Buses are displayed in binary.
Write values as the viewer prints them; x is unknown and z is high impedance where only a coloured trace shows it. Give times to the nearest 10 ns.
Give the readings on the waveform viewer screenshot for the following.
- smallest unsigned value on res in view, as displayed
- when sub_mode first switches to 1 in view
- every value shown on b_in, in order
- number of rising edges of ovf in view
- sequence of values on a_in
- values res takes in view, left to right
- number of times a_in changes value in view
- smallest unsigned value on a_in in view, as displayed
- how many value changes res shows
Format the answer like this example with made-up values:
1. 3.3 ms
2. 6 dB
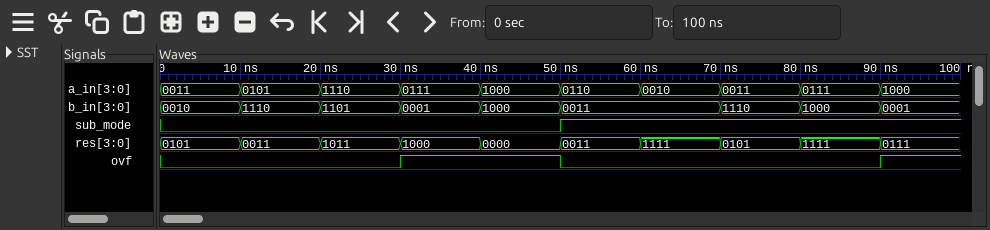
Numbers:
1. 0000
2. 50 ns
3. 0010, 1110, 1101, 0001, 1000, 0011, 1110, 1000, 0001
4. 2
5. 0011, 0101, 1110, 0111, 1000, 0110, 0010, 0011, 0111, 1000
6. 0101, 0011, 1011, 1000, 0000, 0011, 1111, 0101, 1111, 0111
7. 9
8. 0010
9. 9
